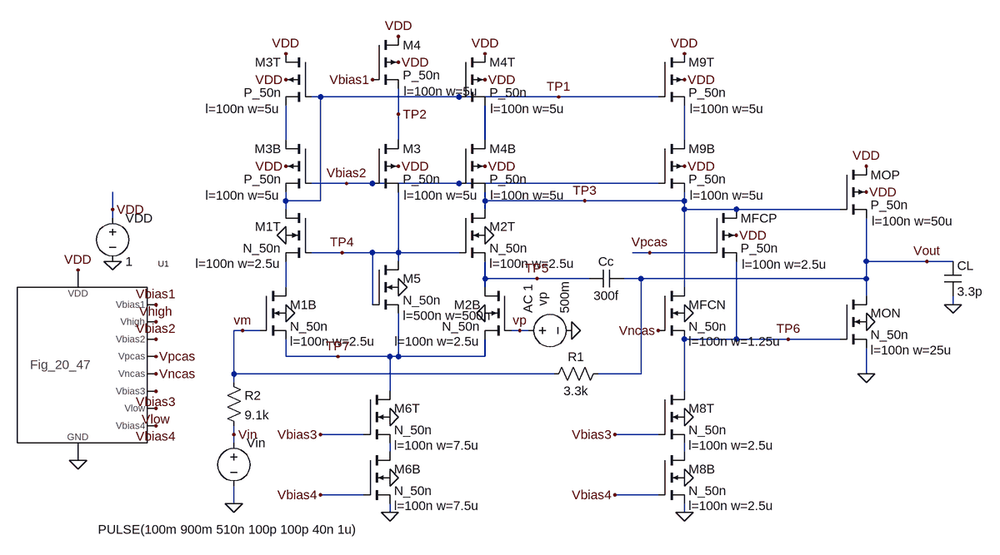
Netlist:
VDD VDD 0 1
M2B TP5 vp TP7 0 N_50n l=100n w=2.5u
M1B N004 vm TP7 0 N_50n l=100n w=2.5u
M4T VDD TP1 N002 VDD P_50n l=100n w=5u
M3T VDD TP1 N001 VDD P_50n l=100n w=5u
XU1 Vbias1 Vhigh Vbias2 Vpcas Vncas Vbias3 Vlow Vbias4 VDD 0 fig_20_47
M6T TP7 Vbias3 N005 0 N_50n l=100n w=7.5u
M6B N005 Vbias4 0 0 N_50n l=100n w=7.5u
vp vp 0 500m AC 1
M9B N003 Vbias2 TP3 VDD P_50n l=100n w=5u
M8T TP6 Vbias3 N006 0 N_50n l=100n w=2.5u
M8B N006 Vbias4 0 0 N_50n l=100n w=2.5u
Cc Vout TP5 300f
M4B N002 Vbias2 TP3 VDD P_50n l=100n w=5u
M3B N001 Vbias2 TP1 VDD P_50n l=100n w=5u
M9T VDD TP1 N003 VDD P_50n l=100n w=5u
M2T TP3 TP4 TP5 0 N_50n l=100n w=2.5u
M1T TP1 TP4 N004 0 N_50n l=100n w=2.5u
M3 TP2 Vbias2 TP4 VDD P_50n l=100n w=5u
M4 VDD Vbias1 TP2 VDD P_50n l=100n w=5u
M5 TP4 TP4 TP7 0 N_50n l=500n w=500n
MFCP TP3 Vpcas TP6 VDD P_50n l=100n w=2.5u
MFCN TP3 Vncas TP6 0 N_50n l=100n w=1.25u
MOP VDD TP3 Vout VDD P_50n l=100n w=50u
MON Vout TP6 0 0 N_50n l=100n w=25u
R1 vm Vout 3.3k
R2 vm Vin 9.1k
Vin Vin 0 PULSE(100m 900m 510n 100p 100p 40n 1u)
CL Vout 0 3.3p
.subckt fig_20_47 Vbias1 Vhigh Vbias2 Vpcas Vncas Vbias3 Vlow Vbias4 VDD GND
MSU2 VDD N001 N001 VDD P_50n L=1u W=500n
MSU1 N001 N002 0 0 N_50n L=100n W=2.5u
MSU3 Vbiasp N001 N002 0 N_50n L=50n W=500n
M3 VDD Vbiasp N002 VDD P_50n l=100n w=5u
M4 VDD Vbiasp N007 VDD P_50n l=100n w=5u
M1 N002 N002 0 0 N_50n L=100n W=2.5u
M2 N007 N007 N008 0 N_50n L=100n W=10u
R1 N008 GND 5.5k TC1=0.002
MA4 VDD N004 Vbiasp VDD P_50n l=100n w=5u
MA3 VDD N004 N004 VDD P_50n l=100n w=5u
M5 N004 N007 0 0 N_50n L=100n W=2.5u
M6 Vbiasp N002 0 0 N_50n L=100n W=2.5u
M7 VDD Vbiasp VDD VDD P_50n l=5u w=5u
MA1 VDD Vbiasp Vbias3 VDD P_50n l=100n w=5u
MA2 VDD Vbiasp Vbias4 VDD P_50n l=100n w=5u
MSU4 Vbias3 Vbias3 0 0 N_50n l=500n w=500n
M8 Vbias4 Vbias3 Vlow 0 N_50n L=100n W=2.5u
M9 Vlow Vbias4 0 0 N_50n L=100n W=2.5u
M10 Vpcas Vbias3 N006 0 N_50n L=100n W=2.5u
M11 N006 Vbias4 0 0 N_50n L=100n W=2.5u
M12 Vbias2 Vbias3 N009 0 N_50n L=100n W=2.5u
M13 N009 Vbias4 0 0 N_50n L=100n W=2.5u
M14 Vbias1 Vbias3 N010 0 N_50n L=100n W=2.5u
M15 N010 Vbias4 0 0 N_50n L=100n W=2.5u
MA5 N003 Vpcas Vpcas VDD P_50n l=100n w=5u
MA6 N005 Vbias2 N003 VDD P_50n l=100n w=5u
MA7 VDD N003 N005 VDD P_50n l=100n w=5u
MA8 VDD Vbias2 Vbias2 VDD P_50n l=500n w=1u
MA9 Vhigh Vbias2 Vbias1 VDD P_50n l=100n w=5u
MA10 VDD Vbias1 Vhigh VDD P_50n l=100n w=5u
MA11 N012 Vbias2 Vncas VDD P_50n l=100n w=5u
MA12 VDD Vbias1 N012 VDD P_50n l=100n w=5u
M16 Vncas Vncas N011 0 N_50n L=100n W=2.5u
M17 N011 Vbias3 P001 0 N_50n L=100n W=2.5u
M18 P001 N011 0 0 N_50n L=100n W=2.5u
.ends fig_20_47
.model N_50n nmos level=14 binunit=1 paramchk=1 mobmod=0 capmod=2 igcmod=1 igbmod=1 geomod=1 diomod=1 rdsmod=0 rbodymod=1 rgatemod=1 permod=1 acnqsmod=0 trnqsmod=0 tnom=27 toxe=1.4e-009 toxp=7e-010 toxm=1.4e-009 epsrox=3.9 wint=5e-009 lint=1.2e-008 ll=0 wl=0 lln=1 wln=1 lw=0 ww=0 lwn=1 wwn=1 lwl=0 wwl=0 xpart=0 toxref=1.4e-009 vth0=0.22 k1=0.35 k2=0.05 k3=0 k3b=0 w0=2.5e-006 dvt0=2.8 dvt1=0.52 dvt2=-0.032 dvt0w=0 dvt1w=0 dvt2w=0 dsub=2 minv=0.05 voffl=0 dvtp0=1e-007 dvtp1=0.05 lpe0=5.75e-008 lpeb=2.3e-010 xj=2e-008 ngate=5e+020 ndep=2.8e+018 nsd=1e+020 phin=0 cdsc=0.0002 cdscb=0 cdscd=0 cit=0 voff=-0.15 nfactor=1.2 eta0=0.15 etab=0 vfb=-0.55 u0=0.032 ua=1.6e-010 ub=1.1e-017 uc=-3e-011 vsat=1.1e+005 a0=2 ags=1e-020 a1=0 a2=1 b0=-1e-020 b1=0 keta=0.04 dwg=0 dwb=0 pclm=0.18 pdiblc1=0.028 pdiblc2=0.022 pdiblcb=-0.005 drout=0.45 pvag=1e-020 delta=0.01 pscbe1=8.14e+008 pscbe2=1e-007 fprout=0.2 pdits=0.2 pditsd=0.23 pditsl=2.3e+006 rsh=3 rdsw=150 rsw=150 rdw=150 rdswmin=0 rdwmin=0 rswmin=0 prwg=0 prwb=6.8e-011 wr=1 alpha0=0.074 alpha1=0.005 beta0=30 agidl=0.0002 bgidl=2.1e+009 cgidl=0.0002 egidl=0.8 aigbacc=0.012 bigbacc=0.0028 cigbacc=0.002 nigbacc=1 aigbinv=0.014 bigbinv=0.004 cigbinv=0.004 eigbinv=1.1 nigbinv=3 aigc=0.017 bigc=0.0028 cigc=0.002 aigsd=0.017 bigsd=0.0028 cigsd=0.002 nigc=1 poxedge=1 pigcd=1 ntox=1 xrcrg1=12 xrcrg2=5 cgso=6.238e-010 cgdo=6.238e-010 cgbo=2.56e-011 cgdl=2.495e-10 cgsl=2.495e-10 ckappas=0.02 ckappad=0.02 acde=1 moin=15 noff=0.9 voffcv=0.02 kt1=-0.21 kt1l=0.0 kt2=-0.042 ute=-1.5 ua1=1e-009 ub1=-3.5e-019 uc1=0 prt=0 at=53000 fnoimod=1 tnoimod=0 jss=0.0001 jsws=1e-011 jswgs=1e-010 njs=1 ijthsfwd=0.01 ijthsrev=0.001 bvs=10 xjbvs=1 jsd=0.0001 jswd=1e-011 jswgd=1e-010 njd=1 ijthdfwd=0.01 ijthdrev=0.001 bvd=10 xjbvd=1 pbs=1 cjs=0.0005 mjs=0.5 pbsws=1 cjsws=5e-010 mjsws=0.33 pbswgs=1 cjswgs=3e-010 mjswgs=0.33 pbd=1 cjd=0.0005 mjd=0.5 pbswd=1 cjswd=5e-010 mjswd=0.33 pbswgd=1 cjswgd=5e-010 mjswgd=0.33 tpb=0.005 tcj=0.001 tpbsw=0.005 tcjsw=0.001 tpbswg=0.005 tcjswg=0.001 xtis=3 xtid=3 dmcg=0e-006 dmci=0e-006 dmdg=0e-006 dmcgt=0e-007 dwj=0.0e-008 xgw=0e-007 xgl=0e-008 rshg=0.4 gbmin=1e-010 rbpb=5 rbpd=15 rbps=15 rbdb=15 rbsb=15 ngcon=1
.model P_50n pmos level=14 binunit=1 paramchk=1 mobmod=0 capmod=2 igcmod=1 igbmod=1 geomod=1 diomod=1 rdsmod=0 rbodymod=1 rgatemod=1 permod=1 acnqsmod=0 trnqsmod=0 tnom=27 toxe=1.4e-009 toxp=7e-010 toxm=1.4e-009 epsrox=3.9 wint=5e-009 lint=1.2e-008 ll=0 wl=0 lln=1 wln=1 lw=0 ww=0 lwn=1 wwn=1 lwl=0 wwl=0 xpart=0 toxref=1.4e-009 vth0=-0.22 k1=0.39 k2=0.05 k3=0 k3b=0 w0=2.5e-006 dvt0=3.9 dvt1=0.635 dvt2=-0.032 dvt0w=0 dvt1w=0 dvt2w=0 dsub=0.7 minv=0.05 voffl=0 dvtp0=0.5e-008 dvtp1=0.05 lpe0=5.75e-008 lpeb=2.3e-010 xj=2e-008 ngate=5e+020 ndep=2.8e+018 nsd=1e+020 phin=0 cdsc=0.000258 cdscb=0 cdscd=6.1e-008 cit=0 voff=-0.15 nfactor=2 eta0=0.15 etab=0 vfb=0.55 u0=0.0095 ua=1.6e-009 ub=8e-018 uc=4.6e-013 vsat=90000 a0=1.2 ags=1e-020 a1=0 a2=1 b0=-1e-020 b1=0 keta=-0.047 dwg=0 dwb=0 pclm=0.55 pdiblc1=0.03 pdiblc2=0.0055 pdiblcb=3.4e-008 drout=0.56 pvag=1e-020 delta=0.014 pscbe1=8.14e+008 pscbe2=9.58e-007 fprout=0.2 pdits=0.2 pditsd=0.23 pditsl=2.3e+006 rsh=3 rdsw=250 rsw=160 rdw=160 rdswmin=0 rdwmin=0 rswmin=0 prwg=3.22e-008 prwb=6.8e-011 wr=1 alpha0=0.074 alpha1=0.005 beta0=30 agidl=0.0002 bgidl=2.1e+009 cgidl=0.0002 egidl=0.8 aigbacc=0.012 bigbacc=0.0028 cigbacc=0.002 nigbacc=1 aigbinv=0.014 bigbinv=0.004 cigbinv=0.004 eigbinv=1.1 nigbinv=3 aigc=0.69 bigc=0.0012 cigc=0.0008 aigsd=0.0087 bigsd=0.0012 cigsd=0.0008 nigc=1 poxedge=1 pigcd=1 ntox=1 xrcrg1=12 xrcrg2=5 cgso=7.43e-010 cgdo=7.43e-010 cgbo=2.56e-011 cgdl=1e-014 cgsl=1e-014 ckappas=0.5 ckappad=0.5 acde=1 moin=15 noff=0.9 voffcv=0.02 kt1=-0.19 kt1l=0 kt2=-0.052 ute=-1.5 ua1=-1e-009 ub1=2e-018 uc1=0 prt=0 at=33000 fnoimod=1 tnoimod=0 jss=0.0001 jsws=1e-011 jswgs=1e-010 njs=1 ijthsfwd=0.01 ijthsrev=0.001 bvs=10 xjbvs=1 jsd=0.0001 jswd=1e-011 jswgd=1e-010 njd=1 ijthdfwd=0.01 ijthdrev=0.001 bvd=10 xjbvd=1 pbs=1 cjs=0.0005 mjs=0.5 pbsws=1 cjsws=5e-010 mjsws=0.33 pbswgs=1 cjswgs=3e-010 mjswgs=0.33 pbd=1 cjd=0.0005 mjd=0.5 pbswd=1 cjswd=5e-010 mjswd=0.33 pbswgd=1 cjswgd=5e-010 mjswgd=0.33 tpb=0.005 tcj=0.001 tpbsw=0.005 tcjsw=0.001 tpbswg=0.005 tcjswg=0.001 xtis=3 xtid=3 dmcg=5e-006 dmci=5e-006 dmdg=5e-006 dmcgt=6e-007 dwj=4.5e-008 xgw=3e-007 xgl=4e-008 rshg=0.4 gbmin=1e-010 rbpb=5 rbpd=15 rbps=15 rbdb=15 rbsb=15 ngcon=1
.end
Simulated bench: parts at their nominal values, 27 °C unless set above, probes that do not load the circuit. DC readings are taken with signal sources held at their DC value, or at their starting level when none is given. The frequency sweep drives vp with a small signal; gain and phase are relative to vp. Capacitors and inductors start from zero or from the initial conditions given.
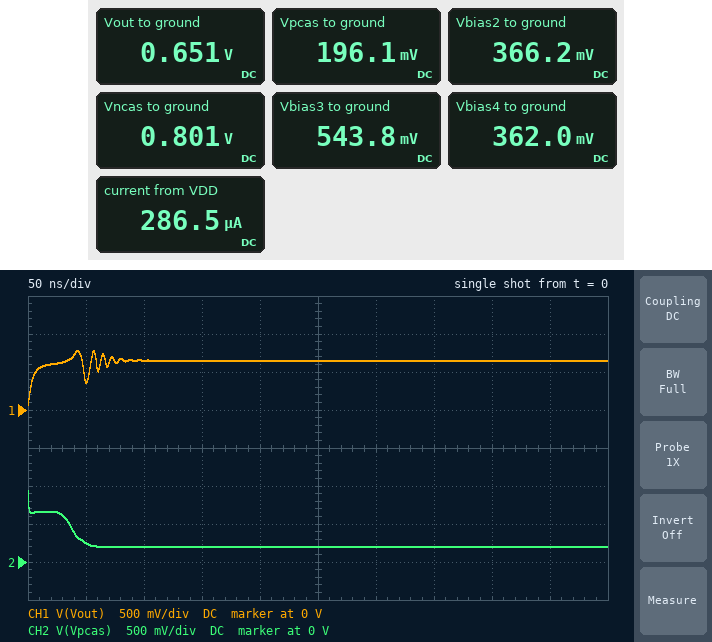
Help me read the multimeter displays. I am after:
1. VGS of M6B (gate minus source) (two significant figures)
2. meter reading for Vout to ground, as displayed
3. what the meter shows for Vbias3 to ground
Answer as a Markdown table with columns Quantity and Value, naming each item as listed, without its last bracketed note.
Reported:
| Quantity | Value |
|---|---|
| VGS of M6B (gate minus source) | 360 mV |
| meter reading for Vout to ground, as displayed | 0.651 V |
| what the meter shows for Vbias3 to ground | 543.8 mV |
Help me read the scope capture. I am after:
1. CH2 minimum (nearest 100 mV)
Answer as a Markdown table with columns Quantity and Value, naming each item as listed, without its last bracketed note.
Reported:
| Quantity | Value |
|---|---|
| CH2 minimum | 200 mV |
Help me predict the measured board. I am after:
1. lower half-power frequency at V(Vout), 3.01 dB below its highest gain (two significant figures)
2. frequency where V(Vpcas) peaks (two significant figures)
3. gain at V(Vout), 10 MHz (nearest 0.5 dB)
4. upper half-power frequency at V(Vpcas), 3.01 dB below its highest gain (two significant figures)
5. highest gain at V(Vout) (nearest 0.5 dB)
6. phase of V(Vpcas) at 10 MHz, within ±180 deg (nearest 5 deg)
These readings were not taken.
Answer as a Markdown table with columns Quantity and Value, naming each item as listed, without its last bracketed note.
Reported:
| Quantity | Value |
|---|---|
| lower half-power frequency at V(Vout), 3.01 dB below its highest gain | 96 MHz |
| frequency where V(Vpcas) peaks | 120 MHz |
| gain at V(Vout), 10 MHz | 2.0 dB |
| upper half-power frequency at V(Vpcas), 3.01 dB below its highest gain | 140 MHz |
| highest gain at V(Vout) | 10.0 dB |
| phase of V(Vpcas) at 10 MHz, within ±180 deg | -90 deg |
